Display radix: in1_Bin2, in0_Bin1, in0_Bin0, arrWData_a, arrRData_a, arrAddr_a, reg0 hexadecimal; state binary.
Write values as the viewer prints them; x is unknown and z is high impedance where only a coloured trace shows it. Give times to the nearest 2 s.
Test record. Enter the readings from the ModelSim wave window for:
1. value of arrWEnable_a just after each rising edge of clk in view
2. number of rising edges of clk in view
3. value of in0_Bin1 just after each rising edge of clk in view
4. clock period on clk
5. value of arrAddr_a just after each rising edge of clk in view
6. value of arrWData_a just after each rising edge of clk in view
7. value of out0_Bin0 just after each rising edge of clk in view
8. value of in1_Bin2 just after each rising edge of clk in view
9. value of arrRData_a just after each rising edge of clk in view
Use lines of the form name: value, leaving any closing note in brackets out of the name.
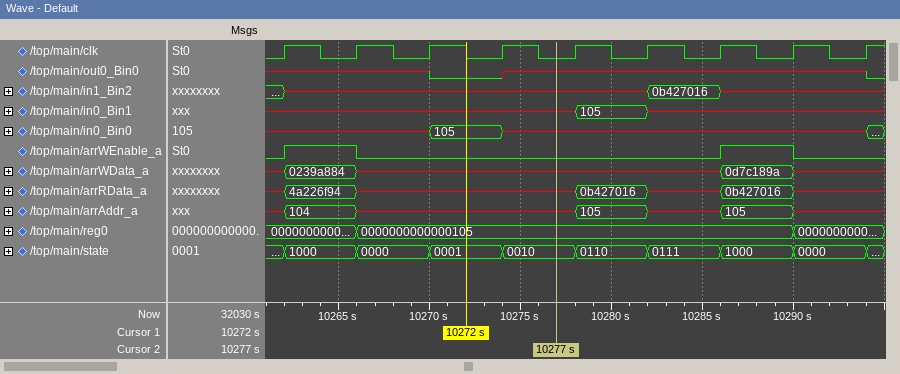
value of arrWEnable_a just after each rising edge of clk in view: 1 0 0 0 0 0 1 0 0
number of rising edges of clk in view: 9
value of in0_Bin1 just after each rising edge of clk in view: x, x, x, x, 105, x, x, x, x
clock period on clk: 4 s
value of arrAddr_a just after each rising edge of clk in view: 104, x, x, x, 105, x, 105, x, x
value of arrWData_a just after each rising edge of clk in view: 0239a884, x, x, x, x, x, 0d7c189a, x, x
value of out0_Bin0 just after each rising edge of clk in view: x x 0 x x x x x 0
value of in1_Bin2 just after each rising edge of clk in view: x, x, x, x, x, 0b427016, x, x, x
value of arrRData_a just after each rising edge of clk in view: 4a226f94, x, x, x, 0b427016, x, 0b427016, x, x
